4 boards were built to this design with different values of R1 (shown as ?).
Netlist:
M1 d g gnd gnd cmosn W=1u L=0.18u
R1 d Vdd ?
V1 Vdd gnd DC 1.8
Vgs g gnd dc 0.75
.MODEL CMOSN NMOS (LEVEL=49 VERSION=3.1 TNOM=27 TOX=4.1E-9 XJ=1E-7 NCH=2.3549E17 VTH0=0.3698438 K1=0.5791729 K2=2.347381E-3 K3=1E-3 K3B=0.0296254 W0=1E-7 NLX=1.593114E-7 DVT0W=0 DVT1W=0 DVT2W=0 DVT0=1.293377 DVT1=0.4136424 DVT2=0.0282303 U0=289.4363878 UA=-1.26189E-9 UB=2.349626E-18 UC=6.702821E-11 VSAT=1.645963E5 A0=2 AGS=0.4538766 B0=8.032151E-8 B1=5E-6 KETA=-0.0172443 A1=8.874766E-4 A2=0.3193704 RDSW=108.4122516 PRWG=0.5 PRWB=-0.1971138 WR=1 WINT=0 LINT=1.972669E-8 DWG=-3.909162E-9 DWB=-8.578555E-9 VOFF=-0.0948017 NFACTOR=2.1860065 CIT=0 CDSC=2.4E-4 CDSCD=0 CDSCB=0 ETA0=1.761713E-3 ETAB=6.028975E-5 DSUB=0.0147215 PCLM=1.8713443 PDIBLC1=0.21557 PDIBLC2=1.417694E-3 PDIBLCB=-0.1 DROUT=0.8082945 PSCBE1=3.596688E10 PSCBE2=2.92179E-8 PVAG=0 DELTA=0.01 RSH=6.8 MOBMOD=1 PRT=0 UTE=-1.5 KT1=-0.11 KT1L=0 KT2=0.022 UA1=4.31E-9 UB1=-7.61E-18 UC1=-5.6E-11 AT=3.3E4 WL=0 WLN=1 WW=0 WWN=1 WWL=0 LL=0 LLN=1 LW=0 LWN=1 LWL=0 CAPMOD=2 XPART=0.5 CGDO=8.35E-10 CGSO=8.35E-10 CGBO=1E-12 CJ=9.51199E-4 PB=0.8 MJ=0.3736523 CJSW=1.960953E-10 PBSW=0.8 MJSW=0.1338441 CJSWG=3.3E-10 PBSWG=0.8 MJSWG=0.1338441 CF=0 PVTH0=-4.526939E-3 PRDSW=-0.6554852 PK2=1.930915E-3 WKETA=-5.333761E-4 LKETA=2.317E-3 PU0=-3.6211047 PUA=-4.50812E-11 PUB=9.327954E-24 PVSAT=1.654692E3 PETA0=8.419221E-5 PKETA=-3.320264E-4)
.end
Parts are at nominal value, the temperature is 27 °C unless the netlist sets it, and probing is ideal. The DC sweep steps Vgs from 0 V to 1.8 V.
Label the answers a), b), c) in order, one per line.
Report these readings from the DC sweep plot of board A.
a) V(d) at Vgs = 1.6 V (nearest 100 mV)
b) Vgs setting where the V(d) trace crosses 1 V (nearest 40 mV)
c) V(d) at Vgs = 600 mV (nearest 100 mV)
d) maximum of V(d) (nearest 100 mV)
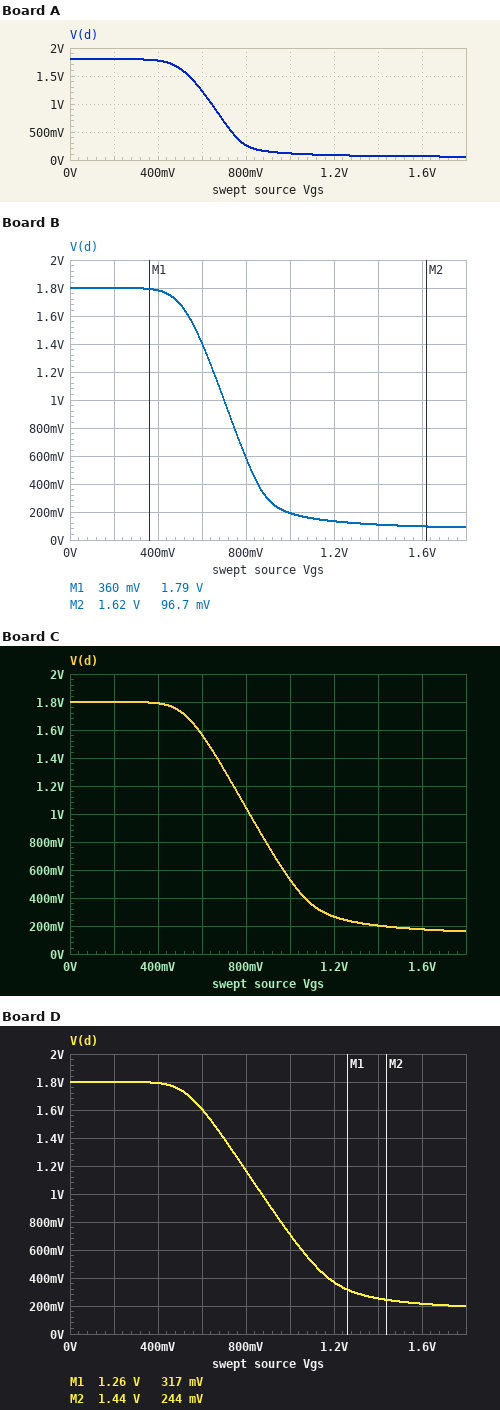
a) 100 mV
b) 640 mV
c) 1.2 V
d) 1.8 V
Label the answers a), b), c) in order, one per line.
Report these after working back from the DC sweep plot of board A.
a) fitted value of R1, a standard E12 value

a) 18 kΩ
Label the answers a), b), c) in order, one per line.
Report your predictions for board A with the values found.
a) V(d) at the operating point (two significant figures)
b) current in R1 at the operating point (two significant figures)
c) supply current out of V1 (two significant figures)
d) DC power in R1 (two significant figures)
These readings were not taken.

a) 430 mV
b) 76 µA
c) 76 µA
d) 100 µW
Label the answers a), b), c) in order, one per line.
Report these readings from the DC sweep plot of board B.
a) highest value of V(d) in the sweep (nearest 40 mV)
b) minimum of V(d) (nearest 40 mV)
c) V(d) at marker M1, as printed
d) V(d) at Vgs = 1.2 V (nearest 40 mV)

a) 1.80 V
b) 80 mV
c) 1.79 V
d) 120 mV
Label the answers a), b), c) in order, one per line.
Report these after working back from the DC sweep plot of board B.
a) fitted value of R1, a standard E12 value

a) 12 kΩ
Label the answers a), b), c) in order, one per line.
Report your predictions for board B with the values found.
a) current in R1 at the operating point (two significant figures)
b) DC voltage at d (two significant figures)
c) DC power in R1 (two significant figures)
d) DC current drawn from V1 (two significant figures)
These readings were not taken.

a) 84 µA
b) 790 mV
c) 85 µW
d) 84 µA
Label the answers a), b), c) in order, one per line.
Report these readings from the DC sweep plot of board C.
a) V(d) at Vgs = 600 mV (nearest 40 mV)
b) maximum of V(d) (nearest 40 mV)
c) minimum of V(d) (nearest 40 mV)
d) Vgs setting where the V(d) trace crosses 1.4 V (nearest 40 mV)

a) 1.56 V
b) 1.80 V
c) 160 mV
d) 680 mV
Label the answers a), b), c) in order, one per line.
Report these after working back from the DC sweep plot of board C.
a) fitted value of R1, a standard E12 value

a) 6.8 kΩ
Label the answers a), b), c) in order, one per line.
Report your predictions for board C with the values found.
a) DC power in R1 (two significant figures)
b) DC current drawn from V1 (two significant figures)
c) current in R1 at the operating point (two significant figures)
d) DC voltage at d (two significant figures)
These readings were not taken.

a) 56 µW
b) 91 µA
c) 91 µA
d) 1.2 V
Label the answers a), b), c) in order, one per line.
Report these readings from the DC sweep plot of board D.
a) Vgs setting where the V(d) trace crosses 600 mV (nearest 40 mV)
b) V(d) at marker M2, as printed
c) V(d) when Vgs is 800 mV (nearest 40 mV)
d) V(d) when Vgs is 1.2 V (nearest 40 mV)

a) 1.04 V
b) 244 mV
c) 1.16 V
d) 360 mV
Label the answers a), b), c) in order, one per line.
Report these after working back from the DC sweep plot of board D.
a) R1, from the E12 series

a) 5.6 kΩ
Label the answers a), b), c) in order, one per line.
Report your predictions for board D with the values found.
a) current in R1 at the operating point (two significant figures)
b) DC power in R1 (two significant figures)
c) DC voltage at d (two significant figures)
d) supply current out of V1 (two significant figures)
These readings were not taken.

a) 92 µA
b) 48 µW
c) 1.3 V
d) 92 µA
